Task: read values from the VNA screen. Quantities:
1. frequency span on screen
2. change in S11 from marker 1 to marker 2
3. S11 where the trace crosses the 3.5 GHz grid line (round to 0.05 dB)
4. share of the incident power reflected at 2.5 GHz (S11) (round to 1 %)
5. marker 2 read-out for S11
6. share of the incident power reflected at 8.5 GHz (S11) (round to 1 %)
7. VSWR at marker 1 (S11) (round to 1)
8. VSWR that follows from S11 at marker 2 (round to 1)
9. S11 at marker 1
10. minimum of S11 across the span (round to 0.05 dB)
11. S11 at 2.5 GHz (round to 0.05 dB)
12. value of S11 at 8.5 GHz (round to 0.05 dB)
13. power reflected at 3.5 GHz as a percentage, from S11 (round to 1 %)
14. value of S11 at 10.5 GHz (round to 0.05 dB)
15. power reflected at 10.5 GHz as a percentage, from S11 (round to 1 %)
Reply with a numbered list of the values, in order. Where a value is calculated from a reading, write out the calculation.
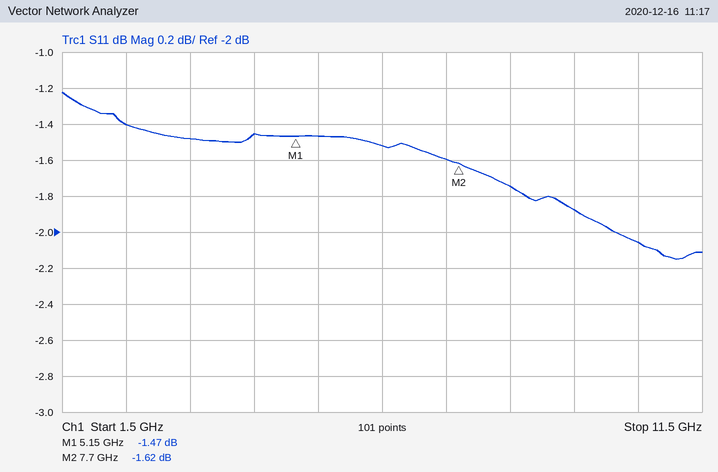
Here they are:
1. 10 GHz
2. -1.62 − (-1.47) = -0.15 dB
3. -1.50 dB
4. 10^(-1.4/10) ≈ 72 %
5. -1.62 dB
6. 10^(-1.75/10) ≈ 67 %
7. (1 + 0.8443)/(1 − 0.8443) ≈ 12
8. (1 + 0.8299)/(1 − 0.8299) ≈ 11
9. -1.47 dB
10. -2.15 dB
11. -1.40 dB
12. -1.75 dB
13. 10^(-1.5/10) ≈ 71 %
14. -2.05 dB
15. 10^(-2.05/10) ≈ 62 %
